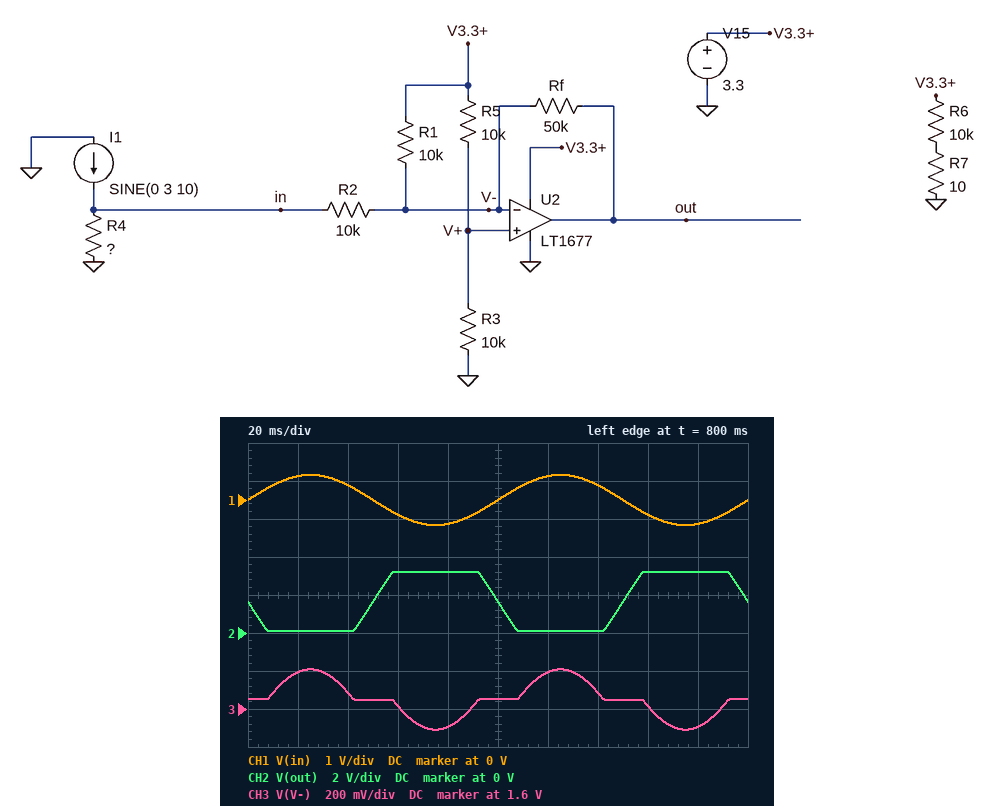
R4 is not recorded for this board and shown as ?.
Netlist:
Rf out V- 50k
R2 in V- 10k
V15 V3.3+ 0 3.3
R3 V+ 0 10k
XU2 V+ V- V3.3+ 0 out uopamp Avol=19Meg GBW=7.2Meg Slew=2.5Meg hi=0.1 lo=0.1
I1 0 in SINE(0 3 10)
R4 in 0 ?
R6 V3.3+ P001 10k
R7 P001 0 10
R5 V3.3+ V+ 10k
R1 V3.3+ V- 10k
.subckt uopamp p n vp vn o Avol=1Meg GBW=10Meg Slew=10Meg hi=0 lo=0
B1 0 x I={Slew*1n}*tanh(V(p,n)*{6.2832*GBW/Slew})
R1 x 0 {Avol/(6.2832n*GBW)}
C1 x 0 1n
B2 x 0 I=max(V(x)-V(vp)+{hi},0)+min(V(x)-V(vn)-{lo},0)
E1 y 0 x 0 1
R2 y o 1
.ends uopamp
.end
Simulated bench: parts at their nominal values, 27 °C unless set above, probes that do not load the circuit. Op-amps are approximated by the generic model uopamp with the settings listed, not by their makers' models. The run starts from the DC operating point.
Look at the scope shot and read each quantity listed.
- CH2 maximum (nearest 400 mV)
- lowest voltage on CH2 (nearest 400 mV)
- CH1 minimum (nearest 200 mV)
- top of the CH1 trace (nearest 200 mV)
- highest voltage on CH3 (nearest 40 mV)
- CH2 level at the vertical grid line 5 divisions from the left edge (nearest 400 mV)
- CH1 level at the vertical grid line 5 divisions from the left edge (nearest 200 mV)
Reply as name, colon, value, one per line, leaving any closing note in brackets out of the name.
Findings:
CH2 maximum: 3.2 V
lowest voltage on CH2: 0 V
CH1 minimum: -600 mV
top of the CH1 trace: 600 mV
highest voltage on CH3: 1.80 V
CH2 level at the vertical grid line 5 divisions from the left edge: 1.6 V
CH1 level at the vertical grid line 5 divisions from the left edge: 0 V
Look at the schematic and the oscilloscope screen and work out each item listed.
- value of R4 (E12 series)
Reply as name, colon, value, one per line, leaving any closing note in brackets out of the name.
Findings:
value of R4: 0.22 Ω
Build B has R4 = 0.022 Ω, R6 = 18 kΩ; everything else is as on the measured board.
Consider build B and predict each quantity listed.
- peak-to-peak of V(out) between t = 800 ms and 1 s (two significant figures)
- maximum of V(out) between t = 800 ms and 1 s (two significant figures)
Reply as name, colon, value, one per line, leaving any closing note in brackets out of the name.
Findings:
peak-to-peak of V(out) between t = 800 ms and 1 s: 660 mV
maximum of V(out) between t = 800 ms and 1 s: 2.0 V
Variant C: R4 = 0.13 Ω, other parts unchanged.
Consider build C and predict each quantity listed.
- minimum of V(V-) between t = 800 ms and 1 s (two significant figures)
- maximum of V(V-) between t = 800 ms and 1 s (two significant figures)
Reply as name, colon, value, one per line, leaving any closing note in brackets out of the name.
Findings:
minimum of V(V-) between t = 800 ms and 1 s: 1.6 V
maximum of V(V-) between t = 800 ms and 1 s: 1.7 V
